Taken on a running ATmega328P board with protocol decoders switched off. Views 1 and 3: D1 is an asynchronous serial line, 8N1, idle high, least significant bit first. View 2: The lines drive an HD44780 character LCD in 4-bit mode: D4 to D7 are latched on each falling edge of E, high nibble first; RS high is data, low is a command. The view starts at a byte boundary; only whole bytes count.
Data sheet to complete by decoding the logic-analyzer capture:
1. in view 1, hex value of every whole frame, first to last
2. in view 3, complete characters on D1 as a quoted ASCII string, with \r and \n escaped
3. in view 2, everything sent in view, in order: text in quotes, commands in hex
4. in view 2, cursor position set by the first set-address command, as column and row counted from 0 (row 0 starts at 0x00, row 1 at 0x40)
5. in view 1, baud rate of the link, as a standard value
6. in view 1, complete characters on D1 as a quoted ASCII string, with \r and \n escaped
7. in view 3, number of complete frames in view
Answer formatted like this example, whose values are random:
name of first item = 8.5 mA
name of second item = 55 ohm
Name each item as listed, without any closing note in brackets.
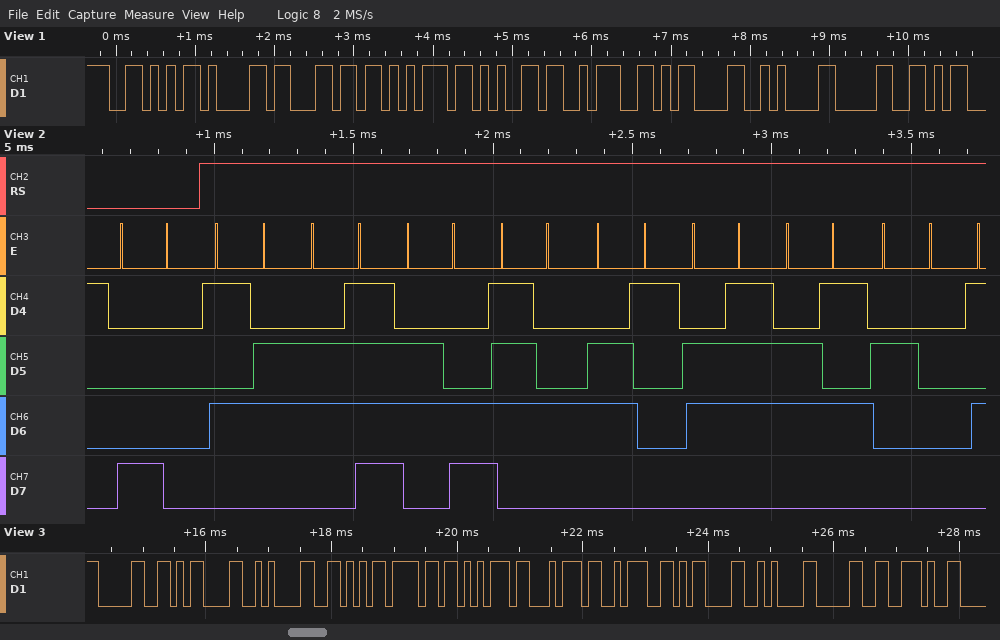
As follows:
in view 1, hex value of every whole frame, first to last = 56 61 6C 75 65 3A 0D 0A 30
in view 3, complete characters on D1 as a quoted ASCII string, with \r and \n escaped = "0\r\nVout:\r\n0."
in view 2, everything sent in view, in order: text in quotes, commands in hex = 0x80 "Voltage "
in view 2, cursor position set by the first set-address command, as column and row counted from 0 = column 0, row 0
in view 1, baud rate of the link, as a standard value = 9600 baud
in view 1, complete characters on D1 as a quoted ASCII string, with \r and \n escaped = "Value:\r\n0"
in view 3, number of complete frames in view = 12
